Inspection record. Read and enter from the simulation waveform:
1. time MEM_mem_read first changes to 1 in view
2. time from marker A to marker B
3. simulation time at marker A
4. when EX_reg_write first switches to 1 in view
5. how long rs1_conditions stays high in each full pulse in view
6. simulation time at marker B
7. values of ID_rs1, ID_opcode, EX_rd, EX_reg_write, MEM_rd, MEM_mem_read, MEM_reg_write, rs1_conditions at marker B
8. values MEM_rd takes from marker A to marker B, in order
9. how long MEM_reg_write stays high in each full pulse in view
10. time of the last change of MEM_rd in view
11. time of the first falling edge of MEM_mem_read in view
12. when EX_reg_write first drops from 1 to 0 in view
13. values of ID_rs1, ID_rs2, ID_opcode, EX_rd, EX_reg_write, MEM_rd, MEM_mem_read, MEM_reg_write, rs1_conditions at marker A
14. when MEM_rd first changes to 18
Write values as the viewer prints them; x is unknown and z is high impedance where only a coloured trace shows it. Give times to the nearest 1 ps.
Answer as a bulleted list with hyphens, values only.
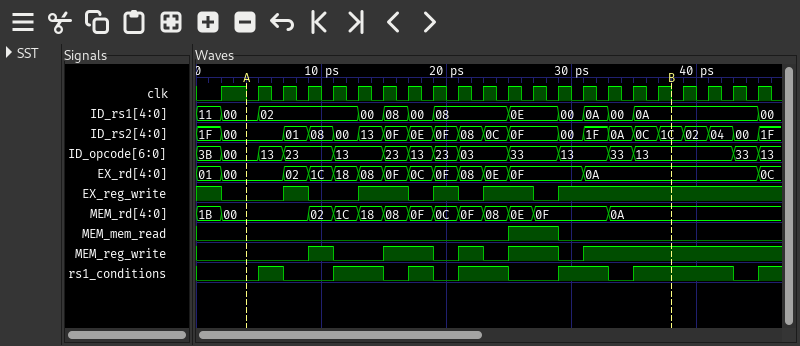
- 25 ps
- 34 ps
- 4 ps
- 7 ps
- 2 ps, 4 ps, 2 ps, 4 ps, 4 ps, 8 ps
- 38 ps
- ID_rs1=0A, ID_opcode=13, EX_rd=0A, EX_reg_write=1, MEM_rd=0A, MEM_mem_read=0, MEM_reg_write=1, rs1_conditions=1
- 00, 02, 1C, 18, 08, 0F, 0C, 0F, 08, 0E, 0F, 0A
- 2 ps, 4 ps, 2 ps, 4 ps
- 33 ps
- 29 ps
- 2 ps
- ID_rs1=00, ID_rs2=00, ID_opcode=00, EX_rd=00, EX_reg_write=0, MEM_rd=00, MEM_mem_read=0, MEM_reg_write=0, rs1_conditions=0
- 13 ps
